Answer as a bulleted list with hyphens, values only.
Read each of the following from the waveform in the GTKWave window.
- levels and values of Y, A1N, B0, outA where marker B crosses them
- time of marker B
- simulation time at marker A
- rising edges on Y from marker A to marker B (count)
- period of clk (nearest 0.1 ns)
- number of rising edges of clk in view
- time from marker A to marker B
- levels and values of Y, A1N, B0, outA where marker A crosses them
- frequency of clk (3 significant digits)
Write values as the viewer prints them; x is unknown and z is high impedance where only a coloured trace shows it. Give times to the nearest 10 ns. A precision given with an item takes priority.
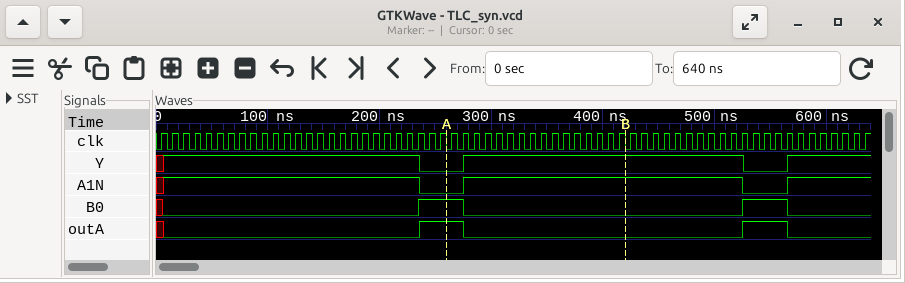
- Y=1, A1N=1, B0=0, outA=0
- 420 ns
- 260 ns
- 1
- 10 ns
- 64
- 160 ns
- Y=0, A1N=0, B0=1, outA=1
- 100 MHz
